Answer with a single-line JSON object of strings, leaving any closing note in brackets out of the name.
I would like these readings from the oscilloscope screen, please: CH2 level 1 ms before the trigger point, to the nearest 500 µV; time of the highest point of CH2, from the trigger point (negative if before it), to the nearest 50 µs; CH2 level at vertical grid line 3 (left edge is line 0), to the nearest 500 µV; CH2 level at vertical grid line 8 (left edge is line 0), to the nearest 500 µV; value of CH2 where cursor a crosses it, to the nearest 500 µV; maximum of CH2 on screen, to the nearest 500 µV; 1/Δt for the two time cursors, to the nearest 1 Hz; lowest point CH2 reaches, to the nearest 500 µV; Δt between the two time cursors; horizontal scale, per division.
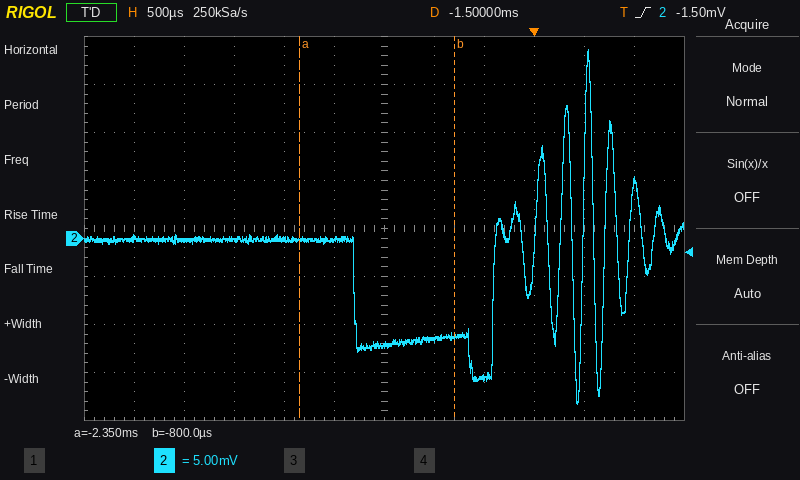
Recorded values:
{"CH2 level 1 ms before the trigger point, to the nearest 500 µV": "-10.5 mV", "time of the highest point of CH2, from the trigger point (negative if before it), to the nearest 50 µs": "+550 µs", "CH2 level at vertical grid line 3 (left edge is line 0), to the nearest 500 µV": "0.0 mV", "CH2 level at vertical grid line 8 (left edge is line 0), to the nearest 500 µV": "-14.5 mV", "value of CH2 where cursor a crosses it, to the nearest 500 µV": "0.0 mV", "maximum of CH2 on screen, to the nearest 500 µV": "19.5 mV", "1/Δt for the two time cursors, to the nearest 1 Hz": "645 Hz", "lowest point CH2 reaches, to the nearest 500 µV": "-17.0 mV", "Δt between the two time cursors": "1.55 ms", "horizontal scale, per division": "500 µs"}
